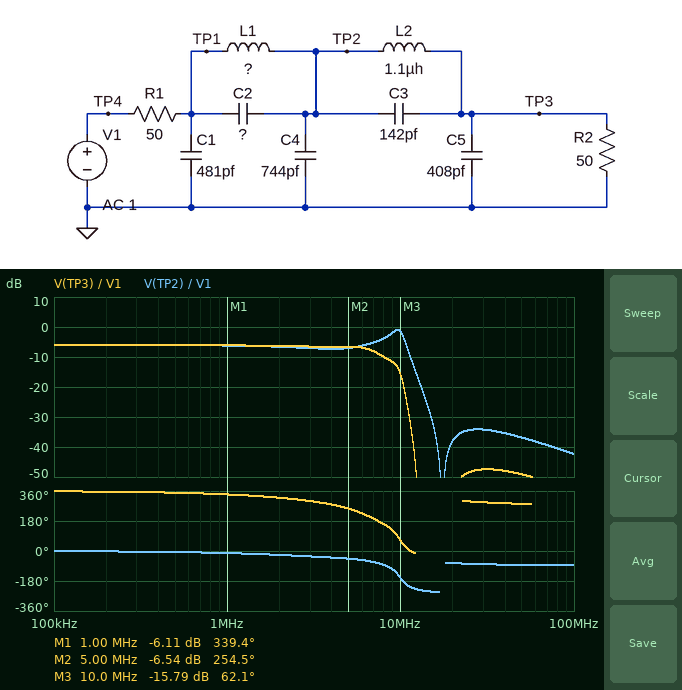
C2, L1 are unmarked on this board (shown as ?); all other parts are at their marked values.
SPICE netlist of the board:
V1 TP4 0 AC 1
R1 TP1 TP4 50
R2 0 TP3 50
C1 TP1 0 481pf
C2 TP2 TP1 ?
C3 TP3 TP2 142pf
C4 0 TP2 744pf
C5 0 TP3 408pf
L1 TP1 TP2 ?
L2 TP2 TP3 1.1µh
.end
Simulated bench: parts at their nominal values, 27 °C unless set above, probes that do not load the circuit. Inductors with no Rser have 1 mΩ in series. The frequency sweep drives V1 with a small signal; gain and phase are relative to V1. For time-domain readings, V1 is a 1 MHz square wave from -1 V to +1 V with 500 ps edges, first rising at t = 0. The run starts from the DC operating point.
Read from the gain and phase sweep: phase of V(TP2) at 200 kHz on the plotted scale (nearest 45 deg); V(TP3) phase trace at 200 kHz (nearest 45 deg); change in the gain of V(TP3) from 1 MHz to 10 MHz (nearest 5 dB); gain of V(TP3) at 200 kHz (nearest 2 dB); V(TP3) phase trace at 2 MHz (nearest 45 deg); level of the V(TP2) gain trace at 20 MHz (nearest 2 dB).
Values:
0 deg
360 deg
-10 dB
-6 dB
315 deg
-38 dB
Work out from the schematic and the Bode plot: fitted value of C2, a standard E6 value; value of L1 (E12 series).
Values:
150 pF
560 nH
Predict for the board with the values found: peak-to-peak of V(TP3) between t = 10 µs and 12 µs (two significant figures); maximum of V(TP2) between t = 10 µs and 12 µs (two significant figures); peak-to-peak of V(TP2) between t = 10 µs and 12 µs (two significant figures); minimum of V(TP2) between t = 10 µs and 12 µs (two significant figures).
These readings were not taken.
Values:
1.2 V
640 mV
1.3 V
-640 mV
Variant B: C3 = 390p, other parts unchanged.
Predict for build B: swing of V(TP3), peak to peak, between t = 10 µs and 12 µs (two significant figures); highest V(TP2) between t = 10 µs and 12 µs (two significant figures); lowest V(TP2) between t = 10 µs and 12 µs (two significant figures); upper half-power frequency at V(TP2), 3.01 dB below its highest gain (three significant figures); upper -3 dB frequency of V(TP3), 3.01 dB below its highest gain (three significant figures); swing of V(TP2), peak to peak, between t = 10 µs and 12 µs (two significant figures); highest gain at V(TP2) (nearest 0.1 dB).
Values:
1.3 V
690 mV
-690 mV
10.1 MHz
5.60 MHz
1.4 V
-3.1 dB
